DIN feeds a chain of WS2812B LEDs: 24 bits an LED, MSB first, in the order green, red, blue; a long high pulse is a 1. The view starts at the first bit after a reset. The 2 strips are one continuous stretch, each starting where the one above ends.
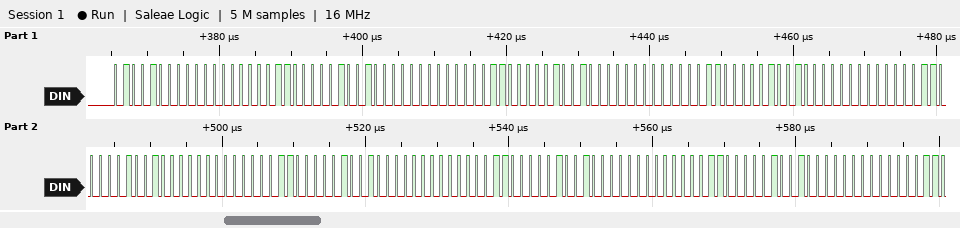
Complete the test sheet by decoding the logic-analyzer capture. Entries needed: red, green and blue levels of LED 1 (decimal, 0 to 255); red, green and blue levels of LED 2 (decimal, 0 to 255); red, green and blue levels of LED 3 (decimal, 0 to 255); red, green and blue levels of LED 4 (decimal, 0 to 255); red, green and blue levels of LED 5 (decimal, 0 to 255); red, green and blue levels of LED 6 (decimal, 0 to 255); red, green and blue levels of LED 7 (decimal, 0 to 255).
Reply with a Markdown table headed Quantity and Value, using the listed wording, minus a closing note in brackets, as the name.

| Quantity | Value |
|---|---|
| red, green and blue levels of LED 1 | 0, 72, 48 |
| red, green and blue levels of LED 2 | 0, 72, 48 |
| red, green and blue levels of LED 3 | 0, 72, 48 |
| red, green and blue levels of LED 4 | 0, 72, 48 |
| red, green and blue levels of LED 5 | 0, 72, 48 |
| red, green and blue levels of LED 6 | 0, 72, 48 |
| red, green and blue levels of LED 7 | 0, 72, 48 |
